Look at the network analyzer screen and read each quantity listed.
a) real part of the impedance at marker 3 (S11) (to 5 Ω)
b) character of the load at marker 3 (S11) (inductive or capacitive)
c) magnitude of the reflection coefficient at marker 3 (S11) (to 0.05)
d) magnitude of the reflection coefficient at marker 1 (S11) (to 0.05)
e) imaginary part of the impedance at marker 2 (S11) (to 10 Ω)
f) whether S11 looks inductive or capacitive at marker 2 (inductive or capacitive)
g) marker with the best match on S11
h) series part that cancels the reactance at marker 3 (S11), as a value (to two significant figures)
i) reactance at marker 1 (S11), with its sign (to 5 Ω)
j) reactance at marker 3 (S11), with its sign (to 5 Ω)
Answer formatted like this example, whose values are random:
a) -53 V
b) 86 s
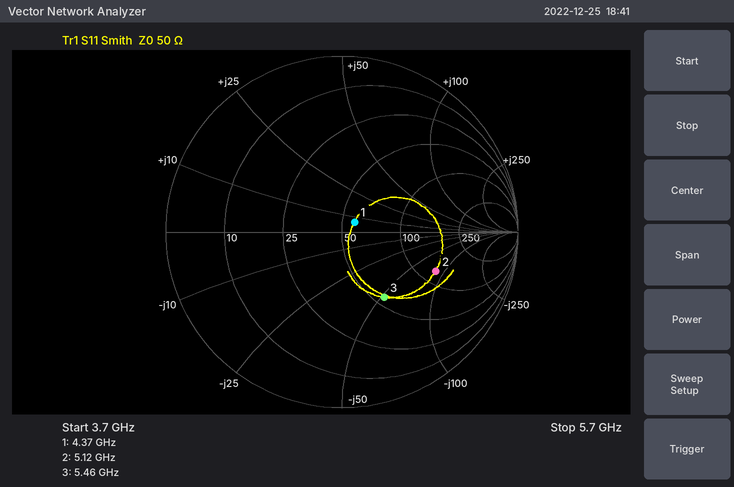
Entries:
a) 55 Ω
b) capacitive
c) 0.45
d) 0.10
e) -80 Ω
f) capacitive
g) marker 1
h) 1.5 nH
i) +5 Ω
j) -50 Ω
